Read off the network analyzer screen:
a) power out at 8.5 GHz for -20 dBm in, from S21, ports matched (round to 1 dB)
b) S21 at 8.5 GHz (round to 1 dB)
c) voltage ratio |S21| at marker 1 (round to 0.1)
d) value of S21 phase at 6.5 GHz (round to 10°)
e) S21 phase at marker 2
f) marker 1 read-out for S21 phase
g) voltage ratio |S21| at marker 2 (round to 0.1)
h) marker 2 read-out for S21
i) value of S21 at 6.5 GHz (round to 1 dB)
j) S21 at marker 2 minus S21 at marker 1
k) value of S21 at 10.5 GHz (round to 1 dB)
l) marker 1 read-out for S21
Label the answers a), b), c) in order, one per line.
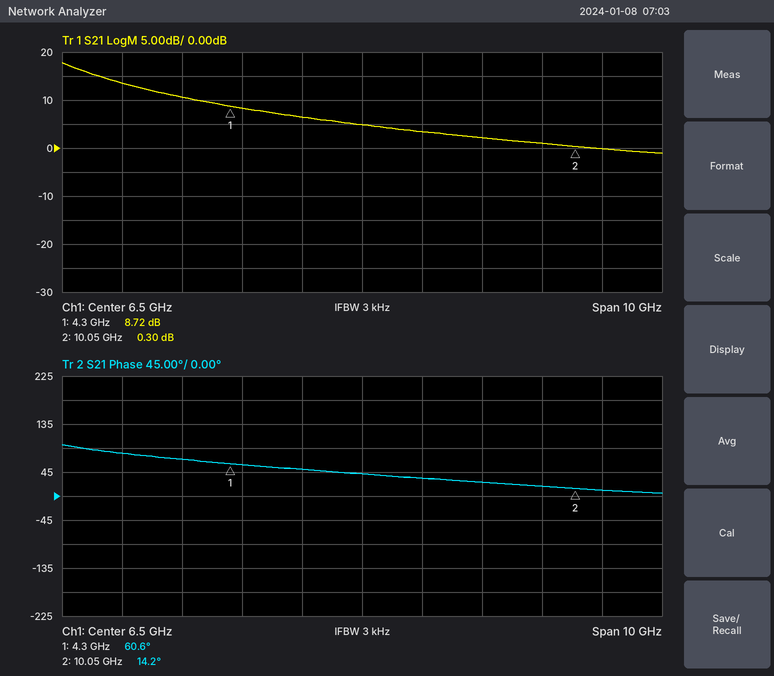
a) -18 dBm
b) 2 dB
c) 2.7
d) 40°
e) 14.2°
f) 60.6°
g) 1.0
h) 0.30 dB
i) 5 dB
j) -8.42 dB
k) 0 dB
l) 8.72 dB
